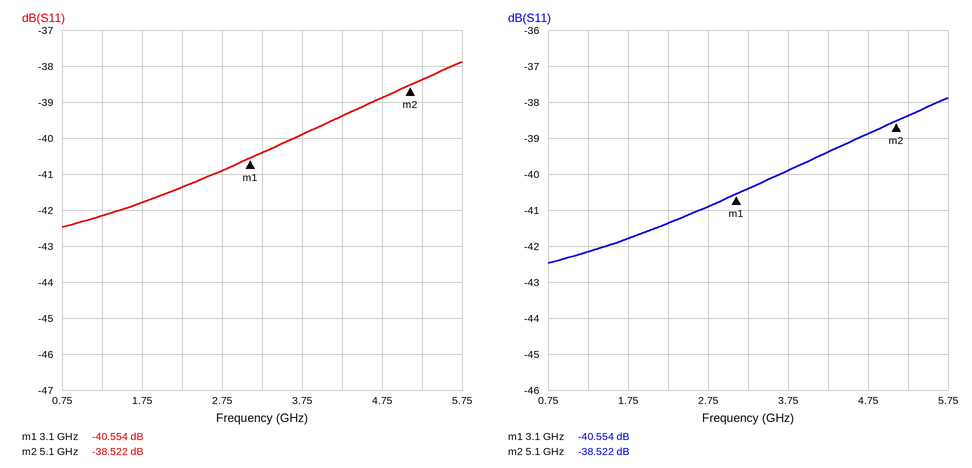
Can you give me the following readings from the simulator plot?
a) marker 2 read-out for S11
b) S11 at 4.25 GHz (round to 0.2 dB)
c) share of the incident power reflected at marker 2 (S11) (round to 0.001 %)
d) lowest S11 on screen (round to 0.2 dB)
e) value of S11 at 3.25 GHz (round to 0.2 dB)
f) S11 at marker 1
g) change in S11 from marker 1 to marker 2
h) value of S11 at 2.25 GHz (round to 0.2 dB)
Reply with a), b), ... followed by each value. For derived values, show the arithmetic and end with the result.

a) -38.522 dB
b) -39.4 dB
c) 10^(-38.522/10) ≈ 0.014 %
d) -42.4 dB
e) -40.4 dB
f) -40.554 dB
g) -38.522 − (-40.554) = 2.032 dB
h) -41.4 dB
